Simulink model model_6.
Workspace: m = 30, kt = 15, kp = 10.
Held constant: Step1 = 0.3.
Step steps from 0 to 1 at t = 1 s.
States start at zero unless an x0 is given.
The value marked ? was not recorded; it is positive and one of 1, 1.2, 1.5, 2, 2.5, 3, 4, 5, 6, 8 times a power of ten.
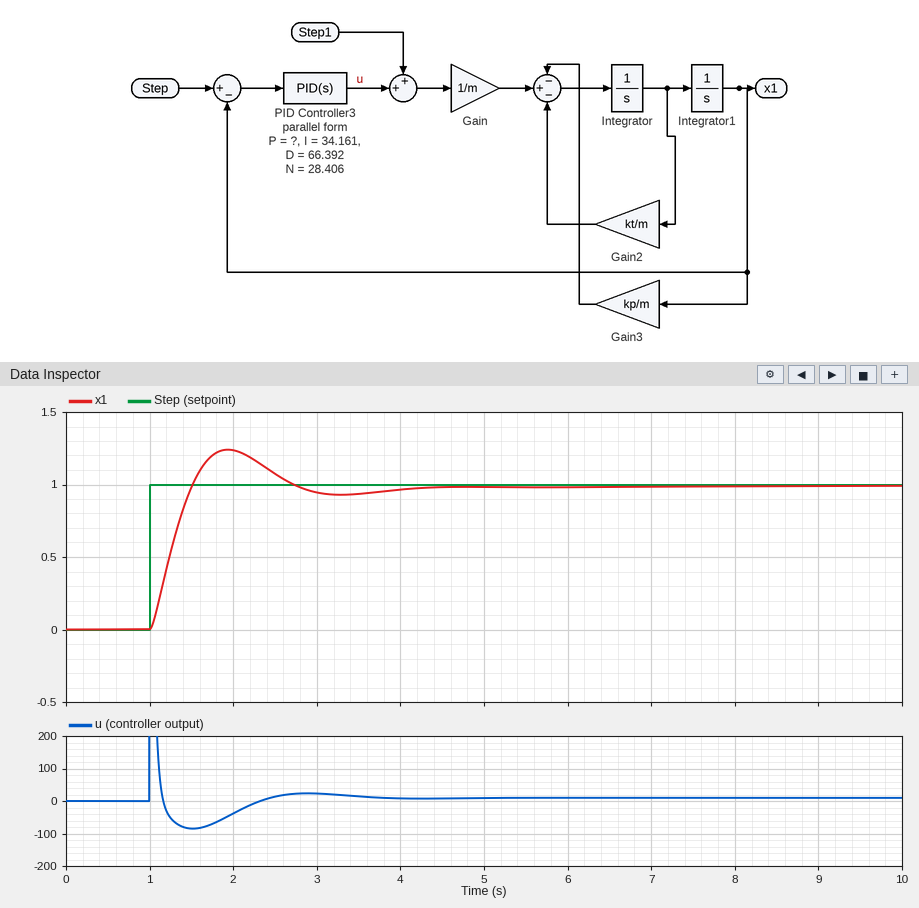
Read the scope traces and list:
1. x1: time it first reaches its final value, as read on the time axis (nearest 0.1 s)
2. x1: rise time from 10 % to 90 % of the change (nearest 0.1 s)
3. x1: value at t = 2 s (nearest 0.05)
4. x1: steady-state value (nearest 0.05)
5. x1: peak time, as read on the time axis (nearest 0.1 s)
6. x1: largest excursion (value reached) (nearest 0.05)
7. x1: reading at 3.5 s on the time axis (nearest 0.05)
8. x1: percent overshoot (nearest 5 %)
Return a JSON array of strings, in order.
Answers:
["1.5 s", "0.4 s", "1.25", "1.00", "1.9 s", "1.25", "0.95", "25 %"]
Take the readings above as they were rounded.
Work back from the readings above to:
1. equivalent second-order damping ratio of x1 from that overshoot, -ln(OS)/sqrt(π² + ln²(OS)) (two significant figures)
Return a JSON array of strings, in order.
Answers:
["0.40"]
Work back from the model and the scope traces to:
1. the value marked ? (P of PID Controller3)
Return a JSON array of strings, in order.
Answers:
["200"]
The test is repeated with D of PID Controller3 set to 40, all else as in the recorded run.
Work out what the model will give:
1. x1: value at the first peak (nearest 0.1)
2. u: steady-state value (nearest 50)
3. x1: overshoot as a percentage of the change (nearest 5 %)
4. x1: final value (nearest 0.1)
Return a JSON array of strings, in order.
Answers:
["1.4", "0", "35 %", "1.0"]
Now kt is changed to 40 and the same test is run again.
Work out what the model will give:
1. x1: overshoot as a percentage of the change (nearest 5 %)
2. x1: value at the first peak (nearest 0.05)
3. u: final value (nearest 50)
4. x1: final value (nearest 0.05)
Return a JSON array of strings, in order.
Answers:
["10 %", "1.10", "0", "1.00"]
